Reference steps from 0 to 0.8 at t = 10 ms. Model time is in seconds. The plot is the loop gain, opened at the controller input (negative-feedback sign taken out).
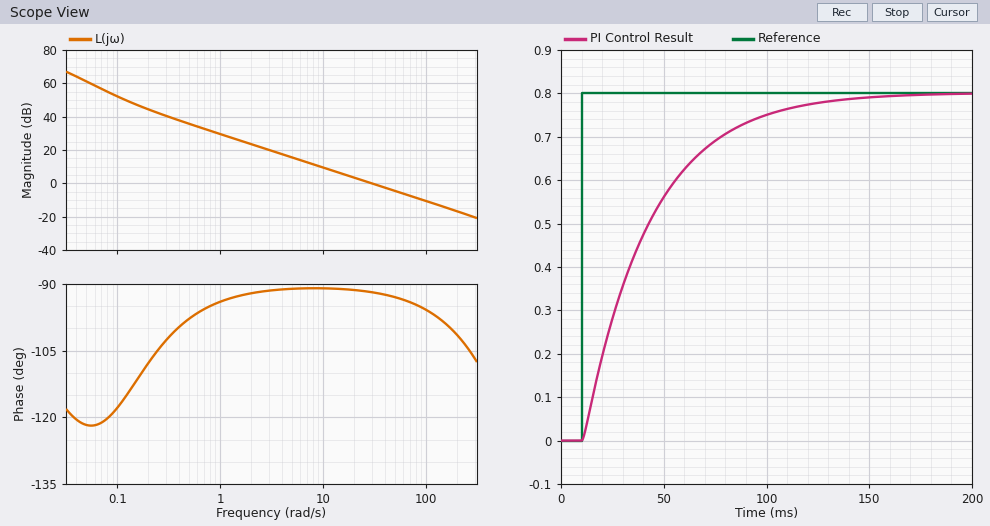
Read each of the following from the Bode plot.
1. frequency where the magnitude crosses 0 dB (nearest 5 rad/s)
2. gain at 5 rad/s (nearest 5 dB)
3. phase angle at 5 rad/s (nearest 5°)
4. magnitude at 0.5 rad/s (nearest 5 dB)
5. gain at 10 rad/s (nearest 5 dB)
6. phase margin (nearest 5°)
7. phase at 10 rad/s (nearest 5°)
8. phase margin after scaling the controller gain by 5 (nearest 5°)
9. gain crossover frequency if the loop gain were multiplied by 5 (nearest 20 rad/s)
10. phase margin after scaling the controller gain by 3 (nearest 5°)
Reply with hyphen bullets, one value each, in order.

- 30 rad/s
- 15 dB
- -90°
- 35 dB
- 10 dB
- 90°
- -90°
- 80°
- 140 rad/s
- 85°
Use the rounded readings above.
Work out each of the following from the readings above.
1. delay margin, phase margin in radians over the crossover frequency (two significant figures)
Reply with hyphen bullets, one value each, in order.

- 0.052 s
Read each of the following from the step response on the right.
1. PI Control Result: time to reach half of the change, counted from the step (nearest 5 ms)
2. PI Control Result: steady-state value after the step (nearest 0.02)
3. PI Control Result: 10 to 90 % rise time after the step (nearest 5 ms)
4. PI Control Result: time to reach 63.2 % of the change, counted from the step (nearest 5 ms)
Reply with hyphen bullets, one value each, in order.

- 25 ms
- 0.80
- 70 ms
- 35 ms
